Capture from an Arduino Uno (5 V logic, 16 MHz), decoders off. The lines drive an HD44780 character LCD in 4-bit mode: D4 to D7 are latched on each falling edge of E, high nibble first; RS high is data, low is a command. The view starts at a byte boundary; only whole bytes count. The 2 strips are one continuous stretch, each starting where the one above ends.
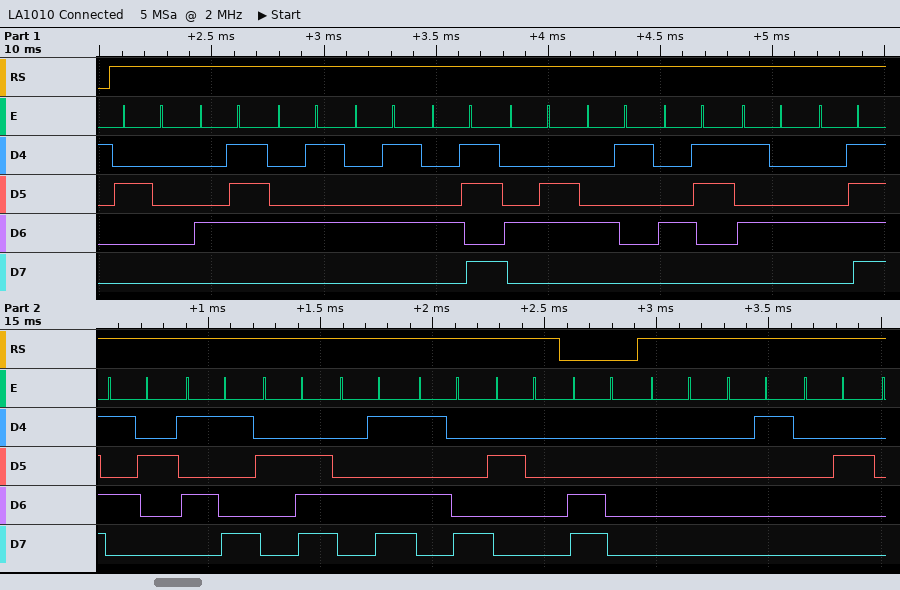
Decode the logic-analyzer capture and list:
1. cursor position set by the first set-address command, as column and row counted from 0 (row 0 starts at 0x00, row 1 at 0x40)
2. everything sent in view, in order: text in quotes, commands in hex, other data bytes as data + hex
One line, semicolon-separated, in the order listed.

column 0, row 1; " GEEKFACTORY.MX " 0xC0 data 00 01 02
